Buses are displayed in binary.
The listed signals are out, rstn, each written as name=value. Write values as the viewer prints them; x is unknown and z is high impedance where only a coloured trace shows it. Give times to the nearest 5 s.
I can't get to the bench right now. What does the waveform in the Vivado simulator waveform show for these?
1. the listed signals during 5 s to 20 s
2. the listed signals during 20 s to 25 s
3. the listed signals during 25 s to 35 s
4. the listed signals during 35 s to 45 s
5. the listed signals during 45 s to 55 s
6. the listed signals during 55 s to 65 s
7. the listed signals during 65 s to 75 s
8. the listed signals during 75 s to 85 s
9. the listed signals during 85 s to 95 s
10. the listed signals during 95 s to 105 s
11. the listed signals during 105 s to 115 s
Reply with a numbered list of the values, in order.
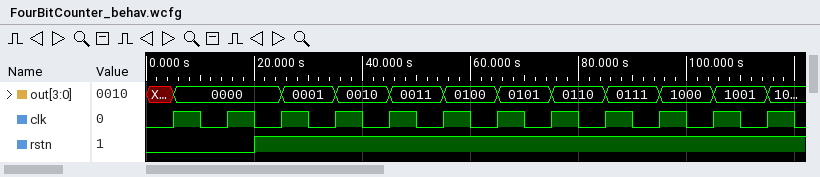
1. out=0000, rstn=0
2. out=0000, rstn=1
3. out=0001, rstn=1
4. out=0010, rstn=1
5. out=0011, rstn=1
6. out=0100, rstn=1
7. out=0101, rstn=1
8. out=0110, rstn=1
9. out=0111, rstn=1
10. out=1000, rstn=1
11. out=1001, rstn=1
